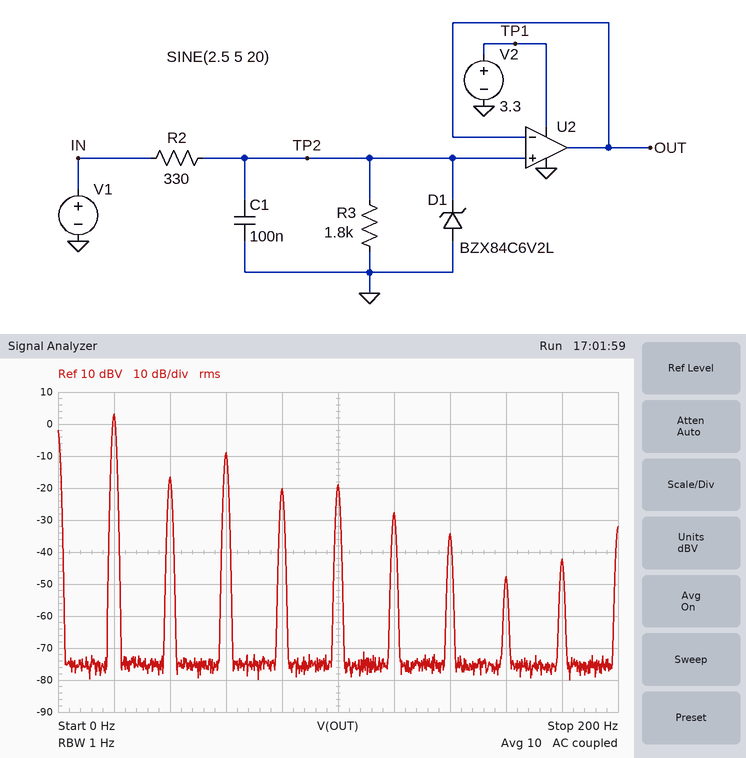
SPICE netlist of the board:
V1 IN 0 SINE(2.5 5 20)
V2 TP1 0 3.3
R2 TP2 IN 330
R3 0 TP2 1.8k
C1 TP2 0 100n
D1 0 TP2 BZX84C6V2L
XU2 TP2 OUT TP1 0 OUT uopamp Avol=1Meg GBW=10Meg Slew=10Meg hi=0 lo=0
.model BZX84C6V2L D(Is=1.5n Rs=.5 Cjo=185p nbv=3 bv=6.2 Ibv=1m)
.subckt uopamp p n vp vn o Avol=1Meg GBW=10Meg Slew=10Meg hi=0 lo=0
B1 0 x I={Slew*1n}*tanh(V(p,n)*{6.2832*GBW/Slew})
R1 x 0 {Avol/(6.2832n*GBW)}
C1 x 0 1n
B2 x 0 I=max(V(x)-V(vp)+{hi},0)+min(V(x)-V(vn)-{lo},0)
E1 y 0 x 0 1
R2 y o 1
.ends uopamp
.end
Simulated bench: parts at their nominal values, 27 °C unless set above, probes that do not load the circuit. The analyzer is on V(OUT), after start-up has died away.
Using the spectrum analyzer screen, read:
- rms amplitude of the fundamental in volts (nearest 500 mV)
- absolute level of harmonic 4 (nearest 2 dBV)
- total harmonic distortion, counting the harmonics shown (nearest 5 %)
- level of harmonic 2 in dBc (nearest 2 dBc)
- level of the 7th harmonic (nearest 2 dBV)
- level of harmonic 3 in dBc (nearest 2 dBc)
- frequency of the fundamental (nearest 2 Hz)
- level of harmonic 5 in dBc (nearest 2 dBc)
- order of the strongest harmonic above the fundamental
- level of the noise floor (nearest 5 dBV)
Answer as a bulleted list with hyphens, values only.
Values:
- 1.5 V
- -20 dBV
- 30 %
- -20 dBc
- -34 dBV
- -12 dBc
- 20 Hz
- -22 dBc
- 3
- -75 dBV
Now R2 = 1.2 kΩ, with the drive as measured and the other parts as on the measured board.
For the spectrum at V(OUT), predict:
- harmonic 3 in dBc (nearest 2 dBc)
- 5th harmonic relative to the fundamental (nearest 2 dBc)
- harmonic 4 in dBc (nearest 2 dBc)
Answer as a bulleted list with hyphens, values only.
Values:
- -14 dBc
- -34 dBc
- -36 dBc
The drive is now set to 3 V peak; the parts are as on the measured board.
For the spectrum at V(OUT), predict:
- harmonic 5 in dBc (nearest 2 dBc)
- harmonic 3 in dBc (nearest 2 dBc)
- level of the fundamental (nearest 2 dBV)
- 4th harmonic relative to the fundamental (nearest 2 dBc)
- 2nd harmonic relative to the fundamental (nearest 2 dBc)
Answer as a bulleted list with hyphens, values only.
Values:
- -54 dBc
- -18 dBc
- 2 dBV
- -36 dBc
- -16 dBc
